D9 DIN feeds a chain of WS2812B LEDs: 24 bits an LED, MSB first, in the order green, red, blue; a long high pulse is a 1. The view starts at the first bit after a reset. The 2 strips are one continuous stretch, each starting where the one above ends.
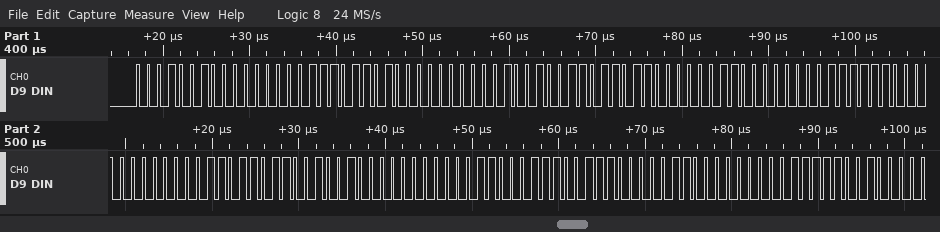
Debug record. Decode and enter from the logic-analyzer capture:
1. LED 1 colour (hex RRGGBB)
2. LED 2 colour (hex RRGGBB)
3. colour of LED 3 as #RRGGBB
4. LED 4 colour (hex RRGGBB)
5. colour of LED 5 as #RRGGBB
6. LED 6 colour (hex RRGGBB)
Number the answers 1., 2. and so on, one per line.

1. #0012ED
2. #2400DB
3. #0003FC
4. #3600C9
5. #1800E7
6. #0006F9
